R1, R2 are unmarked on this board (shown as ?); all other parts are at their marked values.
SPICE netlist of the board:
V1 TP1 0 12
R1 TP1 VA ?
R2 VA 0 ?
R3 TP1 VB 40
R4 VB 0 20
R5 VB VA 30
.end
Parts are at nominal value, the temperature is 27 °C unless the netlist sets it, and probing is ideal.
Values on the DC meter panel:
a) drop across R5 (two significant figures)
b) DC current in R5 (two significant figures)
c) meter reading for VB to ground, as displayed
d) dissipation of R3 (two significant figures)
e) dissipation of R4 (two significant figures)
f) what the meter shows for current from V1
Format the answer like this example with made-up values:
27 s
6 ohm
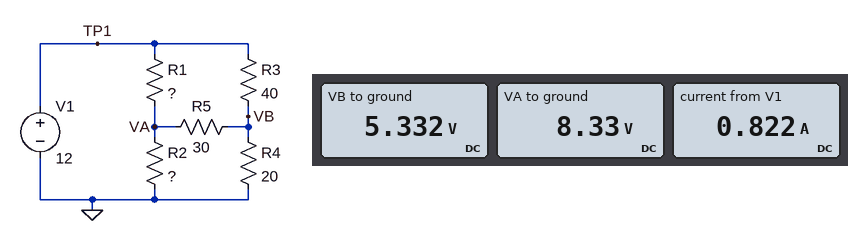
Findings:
3.0 V
100 mA
5.332 V
1.1 W
1.4 W
0.822 A
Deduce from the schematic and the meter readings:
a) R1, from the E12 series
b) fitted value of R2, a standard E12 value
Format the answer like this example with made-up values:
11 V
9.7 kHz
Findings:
5.6 Ω
15 Ω
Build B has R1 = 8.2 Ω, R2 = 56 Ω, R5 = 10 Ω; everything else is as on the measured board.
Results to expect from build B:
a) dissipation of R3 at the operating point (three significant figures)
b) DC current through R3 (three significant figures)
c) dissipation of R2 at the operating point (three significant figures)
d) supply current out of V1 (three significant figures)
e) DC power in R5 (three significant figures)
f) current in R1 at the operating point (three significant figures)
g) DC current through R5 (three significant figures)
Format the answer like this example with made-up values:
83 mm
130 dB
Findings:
669 mW
129 mA
1.43 W
501 mA
450 mW
372 mA
212 mA
